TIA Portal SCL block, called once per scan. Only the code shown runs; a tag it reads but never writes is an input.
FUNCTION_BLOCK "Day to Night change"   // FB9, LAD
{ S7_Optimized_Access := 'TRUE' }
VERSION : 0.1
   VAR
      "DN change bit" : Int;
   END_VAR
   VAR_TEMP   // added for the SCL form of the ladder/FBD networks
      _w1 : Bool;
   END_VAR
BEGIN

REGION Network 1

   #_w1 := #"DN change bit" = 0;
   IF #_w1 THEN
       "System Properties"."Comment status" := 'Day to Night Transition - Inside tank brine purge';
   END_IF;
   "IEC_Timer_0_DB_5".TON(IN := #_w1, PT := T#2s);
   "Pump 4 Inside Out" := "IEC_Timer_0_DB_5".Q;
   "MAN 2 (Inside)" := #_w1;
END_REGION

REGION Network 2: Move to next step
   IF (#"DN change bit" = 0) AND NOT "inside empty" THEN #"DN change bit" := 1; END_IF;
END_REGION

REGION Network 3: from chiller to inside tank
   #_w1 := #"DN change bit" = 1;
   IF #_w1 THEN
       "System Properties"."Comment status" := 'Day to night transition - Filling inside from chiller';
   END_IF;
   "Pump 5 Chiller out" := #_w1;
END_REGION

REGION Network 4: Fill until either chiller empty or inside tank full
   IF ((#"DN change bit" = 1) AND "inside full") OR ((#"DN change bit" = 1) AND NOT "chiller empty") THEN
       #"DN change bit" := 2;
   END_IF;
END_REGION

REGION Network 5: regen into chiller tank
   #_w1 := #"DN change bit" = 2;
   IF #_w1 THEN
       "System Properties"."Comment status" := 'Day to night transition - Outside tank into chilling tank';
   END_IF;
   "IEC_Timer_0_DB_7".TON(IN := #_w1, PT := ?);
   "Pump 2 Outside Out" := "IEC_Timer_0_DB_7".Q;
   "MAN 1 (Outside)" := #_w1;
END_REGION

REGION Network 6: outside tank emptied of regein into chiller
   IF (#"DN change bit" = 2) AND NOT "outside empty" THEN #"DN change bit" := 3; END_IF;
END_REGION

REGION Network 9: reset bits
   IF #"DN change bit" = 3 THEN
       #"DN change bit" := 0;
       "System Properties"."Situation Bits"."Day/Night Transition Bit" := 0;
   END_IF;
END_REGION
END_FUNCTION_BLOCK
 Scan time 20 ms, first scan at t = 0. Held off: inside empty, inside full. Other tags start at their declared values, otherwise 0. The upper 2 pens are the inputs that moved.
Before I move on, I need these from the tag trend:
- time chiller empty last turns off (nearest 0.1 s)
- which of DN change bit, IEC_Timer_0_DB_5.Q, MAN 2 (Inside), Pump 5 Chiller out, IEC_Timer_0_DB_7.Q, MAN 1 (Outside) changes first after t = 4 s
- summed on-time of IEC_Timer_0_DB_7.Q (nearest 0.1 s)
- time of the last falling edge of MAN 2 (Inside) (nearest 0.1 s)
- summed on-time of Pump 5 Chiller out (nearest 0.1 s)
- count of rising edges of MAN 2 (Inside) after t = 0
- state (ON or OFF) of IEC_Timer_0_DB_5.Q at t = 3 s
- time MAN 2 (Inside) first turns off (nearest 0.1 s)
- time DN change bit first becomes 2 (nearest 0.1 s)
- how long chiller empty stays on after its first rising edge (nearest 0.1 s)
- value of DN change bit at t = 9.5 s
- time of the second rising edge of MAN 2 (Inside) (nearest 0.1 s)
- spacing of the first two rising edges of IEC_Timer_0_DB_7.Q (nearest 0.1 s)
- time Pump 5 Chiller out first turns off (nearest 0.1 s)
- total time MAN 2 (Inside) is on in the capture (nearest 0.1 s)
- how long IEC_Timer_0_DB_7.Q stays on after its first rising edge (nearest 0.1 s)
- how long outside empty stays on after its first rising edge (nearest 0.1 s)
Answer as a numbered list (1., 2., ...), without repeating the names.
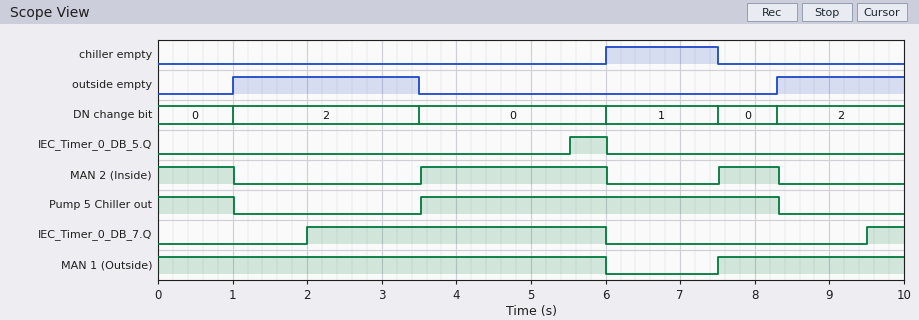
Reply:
1. 7.5 s
2. IEC_Timer_0_DB_5.Q
3. 4.5 s
4. 8.3 s
5. 5.8 s
6. 2
7. OFF
8. 1.0 s
9. 1.0 s
10. 1.5 s
11. 2
12. 7.5 s
13. 7.5 s
14. 1.0 s
15. 4.3 s
16. 4.0 s
17. 2.5 s
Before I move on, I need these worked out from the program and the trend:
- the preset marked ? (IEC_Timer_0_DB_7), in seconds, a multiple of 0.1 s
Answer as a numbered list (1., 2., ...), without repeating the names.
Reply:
1. 2.0 s
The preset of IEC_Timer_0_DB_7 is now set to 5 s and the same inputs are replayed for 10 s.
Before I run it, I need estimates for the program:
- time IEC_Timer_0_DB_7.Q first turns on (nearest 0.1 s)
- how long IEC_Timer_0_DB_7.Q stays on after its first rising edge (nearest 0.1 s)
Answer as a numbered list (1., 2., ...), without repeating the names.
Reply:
1. 5.0 s
2. 1.0 s
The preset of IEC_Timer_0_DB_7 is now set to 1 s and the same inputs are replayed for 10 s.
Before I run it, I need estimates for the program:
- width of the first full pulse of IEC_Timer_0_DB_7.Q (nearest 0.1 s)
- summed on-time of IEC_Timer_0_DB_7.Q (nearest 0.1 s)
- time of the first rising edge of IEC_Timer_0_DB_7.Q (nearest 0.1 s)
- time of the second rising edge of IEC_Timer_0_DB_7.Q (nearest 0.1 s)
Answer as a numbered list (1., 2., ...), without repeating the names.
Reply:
1. 5.0 s
2. 6.5 s
3. 1.0 s
4. 8.5 s
